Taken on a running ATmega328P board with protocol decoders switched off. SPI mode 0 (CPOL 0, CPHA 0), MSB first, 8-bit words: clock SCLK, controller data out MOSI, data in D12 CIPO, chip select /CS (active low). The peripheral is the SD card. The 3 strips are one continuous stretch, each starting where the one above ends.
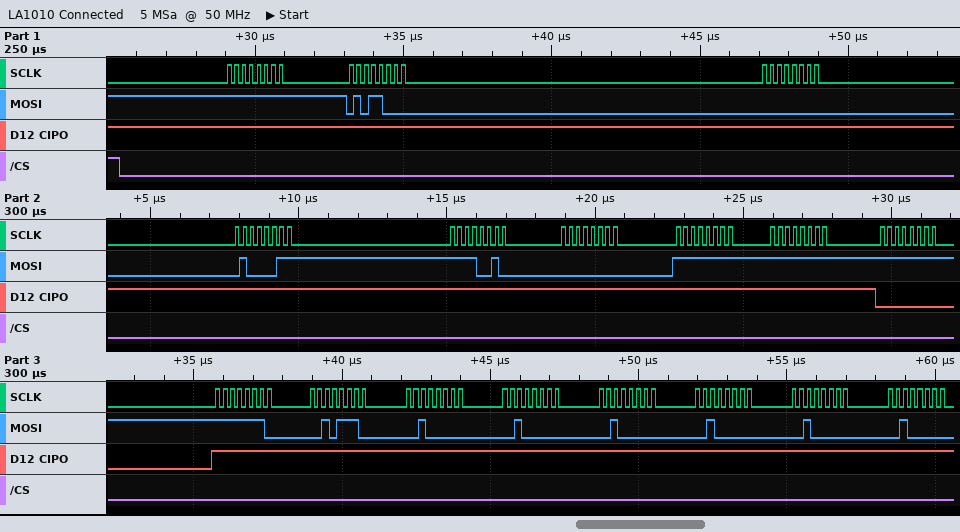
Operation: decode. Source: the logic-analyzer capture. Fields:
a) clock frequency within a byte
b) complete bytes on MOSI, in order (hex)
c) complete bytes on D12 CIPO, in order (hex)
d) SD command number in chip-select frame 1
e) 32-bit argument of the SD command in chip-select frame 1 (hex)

4 MHz
FF 58 00 43 F2 00 FF FF FF FE 2E 20 20 20 20 20 20
FF FF FF FF FF FF FF FF 00 FF FF FF FF FF FF FF FF
CMD24
0x0043F200
